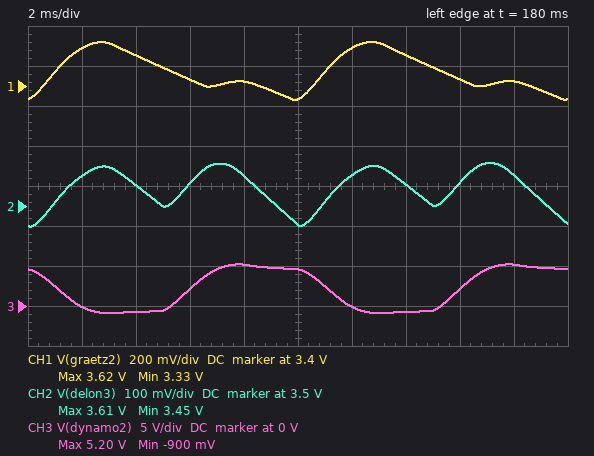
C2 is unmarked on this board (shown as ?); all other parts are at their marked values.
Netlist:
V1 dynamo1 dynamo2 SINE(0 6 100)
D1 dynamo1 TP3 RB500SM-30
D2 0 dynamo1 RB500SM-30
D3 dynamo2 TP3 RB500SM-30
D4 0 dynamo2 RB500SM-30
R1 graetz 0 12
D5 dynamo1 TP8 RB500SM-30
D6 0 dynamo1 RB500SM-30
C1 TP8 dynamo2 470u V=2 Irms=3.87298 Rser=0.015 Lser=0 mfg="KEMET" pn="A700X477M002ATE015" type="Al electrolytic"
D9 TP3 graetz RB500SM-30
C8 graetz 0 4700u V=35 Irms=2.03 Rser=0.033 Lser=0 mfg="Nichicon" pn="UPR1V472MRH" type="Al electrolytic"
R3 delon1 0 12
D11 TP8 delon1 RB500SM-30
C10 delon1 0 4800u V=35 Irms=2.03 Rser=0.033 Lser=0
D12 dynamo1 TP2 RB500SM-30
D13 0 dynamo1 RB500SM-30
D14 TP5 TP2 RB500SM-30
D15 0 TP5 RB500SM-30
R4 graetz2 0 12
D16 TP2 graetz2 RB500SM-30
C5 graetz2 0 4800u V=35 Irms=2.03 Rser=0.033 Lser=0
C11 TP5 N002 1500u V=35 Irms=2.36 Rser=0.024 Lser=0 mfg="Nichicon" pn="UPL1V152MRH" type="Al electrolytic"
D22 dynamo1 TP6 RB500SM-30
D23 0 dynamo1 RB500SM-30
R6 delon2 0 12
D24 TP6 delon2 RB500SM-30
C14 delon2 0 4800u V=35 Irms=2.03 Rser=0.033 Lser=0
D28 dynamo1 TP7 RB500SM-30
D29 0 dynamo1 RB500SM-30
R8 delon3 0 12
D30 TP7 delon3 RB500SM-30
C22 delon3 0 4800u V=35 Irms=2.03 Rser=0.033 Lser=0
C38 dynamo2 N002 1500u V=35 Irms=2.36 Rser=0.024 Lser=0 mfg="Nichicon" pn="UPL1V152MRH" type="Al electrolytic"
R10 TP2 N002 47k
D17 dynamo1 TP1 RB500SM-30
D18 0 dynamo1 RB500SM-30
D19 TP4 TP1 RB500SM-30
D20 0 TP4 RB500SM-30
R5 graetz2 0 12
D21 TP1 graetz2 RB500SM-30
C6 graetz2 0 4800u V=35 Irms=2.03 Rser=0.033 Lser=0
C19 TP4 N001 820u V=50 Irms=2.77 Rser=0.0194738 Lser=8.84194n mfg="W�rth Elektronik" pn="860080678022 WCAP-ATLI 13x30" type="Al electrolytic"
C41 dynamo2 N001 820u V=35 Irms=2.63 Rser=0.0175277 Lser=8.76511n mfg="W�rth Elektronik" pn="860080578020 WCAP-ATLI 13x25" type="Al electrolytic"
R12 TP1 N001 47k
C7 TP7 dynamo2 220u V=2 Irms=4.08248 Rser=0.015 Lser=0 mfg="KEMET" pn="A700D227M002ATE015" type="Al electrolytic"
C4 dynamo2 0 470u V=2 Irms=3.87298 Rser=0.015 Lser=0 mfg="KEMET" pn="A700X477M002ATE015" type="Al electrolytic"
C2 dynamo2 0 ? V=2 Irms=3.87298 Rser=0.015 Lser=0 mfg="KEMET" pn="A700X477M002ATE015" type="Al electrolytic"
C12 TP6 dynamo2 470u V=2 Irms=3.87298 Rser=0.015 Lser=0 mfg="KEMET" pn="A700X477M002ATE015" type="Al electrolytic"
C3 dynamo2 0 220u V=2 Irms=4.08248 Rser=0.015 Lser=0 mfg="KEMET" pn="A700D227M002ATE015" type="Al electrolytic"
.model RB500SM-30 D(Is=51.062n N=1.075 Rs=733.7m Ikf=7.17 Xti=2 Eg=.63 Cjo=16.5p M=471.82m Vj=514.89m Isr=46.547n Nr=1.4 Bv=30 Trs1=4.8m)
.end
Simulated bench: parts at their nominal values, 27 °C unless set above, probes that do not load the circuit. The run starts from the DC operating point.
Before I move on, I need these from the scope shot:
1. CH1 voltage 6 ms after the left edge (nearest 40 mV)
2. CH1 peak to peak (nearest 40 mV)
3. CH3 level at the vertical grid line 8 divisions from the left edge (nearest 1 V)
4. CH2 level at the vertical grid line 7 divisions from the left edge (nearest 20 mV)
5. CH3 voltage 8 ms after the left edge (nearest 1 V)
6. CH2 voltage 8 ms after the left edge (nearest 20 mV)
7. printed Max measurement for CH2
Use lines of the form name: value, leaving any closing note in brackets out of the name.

CH1 voltage 6 ms after the left edge: 3.44 V
CH1 peak to peak: 280 mV
CH3 level at the vertical grid line 8 divisions from the left edge: 2 V
CH2 level at the vertical grid line 7 divisions from the left edge: 3.56 V
CH3 voltage 8 ms after the left edge: 5 V
CH2 voltage 8 ms after the left edge: 3.58 V
printed Max measurement for CH2: 3.61 V
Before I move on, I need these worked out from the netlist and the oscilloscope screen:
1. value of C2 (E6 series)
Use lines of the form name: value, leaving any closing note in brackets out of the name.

value of C2: 680 µF
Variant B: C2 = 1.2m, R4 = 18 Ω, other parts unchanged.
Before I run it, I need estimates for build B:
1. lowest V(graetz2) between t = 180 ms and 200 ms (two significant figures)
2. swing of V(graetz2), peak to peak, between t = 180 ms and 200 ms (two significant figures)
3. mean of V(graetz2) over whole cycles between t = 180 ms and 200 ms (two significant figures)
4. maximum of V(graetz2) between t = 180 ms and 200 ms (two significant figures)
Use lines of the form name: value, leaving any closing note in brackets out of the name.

lowest V(graetz2) between t = 180 ms and 200 ms: 3.7 V
swing of V(graetz2), peak to peak, between t = 180 ms and 200 ms: 330 mV
mean of V(graetz2) over whole cycles between t = 180 ms and 200 ms: 3.9 V
maximum of V(graetz2) between t = 180 ms and 200 ms: 4.1 V
